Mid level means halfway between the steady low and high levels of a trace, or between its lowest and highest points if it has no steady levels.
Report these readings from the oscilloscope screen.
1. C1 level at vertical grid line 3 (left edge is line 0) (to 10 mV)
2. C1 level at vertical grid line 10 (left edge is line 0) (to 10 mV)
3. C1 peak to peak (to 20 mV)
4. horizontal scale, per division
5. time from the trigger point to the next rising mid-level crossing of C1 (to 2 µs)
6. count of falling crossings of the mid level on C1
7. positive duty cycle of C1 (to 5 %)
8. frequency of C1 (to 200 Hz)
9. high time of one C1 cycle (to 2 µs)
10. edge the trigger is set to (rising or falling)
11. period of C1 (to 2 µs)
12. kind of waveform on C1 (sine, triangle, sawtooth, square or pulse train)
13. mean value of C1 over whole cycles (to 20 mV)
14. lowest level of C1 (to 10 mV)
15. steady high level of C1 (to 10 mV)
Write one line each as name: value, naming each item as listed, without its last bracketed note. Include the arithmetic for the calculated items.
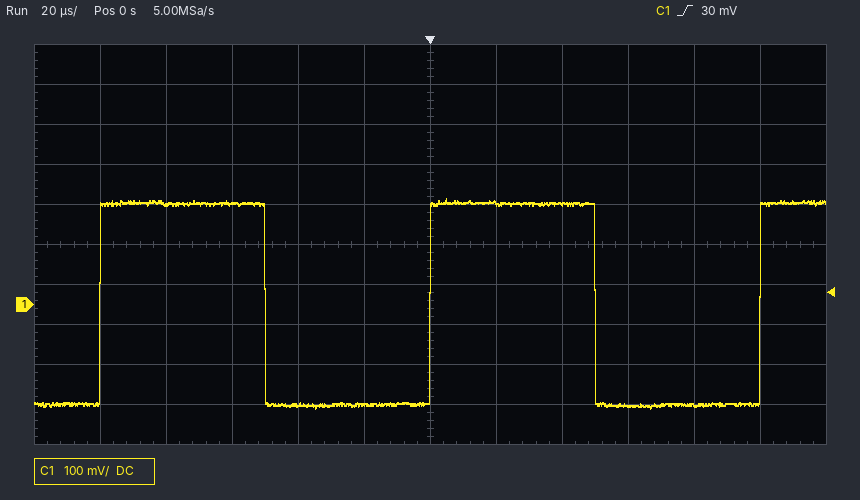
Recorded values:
C1 level at vertical grid line 3 (left edge is line 0): 250 mV
C1 level at vertical grid line 10 (left edge is line 0): -250 mV
C1 peak to peak: 520 mV
horizontal scale, per division: 20 µs
time from the trigger point to the next rising mid-level crossing of C1: 100 µs
count of falling crossings of the mid level on C1: 2
positive duty cycle of C1: 50 µs / 100 µs ≈ 50 %
frequency of C1: 1 / 100 µs ≈ 10.0 kHz
high time of one C1 cycle: 50 µs
edge the trigger is set to: rising
period of C1: 100 µs
kind of waveform on C1: square
mean value of C1 over whole cycles: -260 mV + 0.5 × (250 mV − (-260 mV)) ≈ 0 mV
lowest level of C1: -260 mV
steady high level of C1: 250 mV
